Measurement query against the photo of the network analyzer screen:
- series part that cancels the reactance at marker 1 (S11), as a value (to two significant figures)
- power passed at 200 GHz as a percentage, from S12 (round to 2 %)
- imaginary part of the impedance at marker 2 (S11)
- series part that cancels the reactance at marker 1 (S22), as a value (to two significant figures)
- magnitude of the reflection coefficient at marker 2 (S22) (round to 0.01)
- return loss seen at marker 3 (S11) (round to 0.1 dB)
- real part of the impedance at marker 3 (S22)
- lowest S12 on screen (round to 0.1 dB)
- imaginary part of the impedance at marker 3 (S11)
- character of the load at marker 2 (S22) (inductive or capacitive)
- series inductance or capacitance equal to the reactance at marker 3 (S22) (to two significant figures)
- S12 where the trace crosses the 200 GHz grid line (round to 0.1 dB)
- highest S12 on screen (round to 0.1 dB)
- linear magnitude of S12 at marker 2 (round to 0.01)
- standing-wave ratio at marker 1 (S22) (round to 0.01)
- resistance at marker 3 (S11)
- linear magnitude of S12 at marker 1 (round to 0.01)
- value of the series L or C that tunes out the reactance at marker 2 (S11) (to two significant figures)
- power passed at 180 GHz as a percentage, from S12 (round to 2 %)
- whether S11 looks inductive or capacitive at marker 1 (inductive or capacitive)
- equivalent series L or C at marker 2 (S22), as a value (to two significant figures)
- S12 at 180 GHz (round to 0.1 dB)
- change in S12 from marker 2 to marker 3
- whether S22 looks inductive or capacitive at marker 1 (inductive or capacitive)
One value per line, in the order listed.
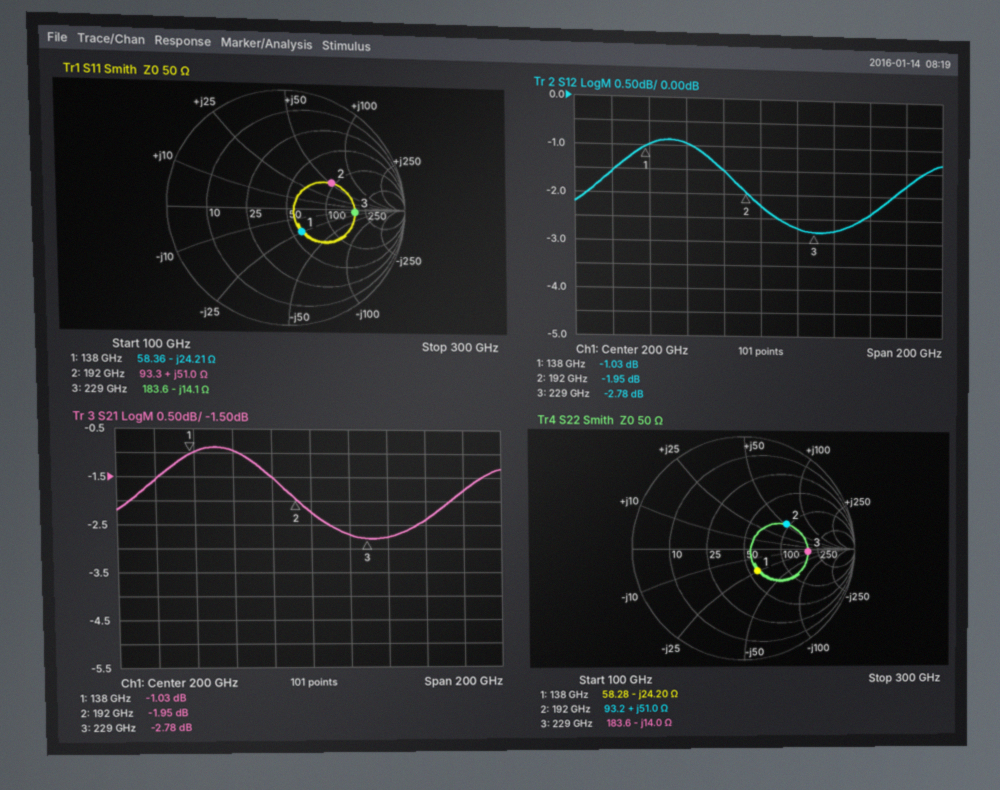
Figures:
28 pH
60 %
+51.0 Ω
28 pH
0.44
4.8 dB
183.6 Ω
-2.8 dB
-14.1 Ω
inductive
50 fF
-2.2 dB
-0.9 dB
0.80
1.60
183.6 Ω
0.89
16 fF
70 %
capacitive
42 pH
-1.5 dB
-0.83 dB
capacitive
